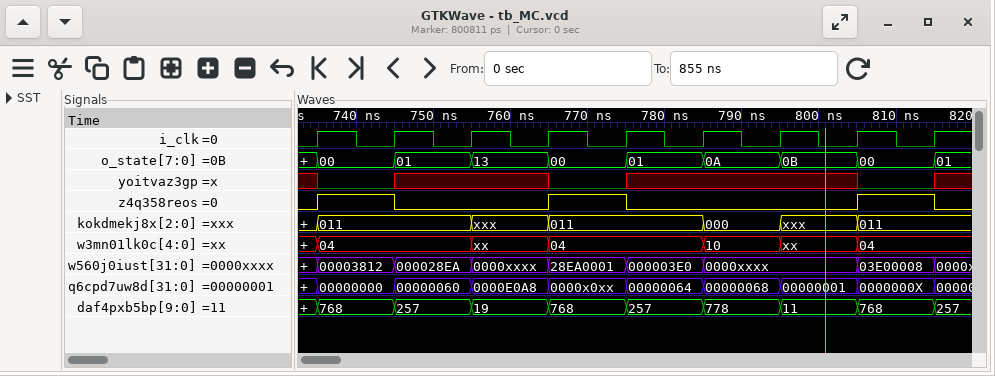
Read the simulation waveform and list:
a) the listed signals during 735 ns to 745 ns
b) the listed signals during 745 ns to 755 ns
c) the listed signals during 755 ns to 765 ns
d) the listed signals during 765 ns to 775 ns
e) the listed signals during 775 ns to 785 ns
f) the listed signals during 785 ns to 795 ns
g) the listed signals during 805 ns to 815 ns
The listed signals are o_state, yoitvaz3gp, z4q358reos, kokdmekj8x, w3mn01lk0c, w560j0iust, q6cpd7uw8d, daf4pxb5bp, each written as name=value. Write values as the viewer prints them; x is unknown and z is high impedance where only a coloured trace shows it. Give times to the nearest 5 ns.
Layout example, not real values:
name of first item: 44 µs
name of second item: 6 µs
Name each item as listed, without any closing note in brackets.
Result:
the listed signals during 735 ns to 745 ns: o_state=00, yoitvaz3gp=0, z4q358reos=1, kokdmekj8x=011, w3mn01lk0c=04, w560j0iust=00003812, q6cpd7uw8d=00000000, daf4pxb5bp=768
the listed signals during 745 ns to 755 ns: o_state=01, yoitvaz3gp=x, z4q358reos=0, kokdmekj8x=011, w3mn01lk0c=04, w560j0iust=000028EA, q6cpd7uw8d=00000060, daf4pxb5bp=257
the listed signals during 755 ns to 765 ns: o_state=13, yoitvaz3gp=x, z4q358reos=0, kokdmekj8x=xxx, w3mn01lk0c=xx, w560j0iust=0000xxxx, q6cpd7uw8d=0000E0A8, daf4pxb5bp=19
the listed signals during 765 ns to 775 ns: o_state=00, yoitvaz3gp=0, z4q358reos=1, kokdmekj8x=011, w3mn01lk0c=04, w560j0iust=28EA0001, q6cpd7uw8d=0000x0xx, daf4pxb5bp=768
the listed signals during 775 ns to 785 ns: o_state=01, yoitvaz3gp=x, z4q358reos=0, kokdmekj8x=011, w3mn01lk0c=04, w560j0iust=000003E0, q6cpd7uw8d=00000064, daf4pxb5bp=257
the listed signals during 785 ns to 795 ns: o_state=0A, yoitvaz3gp=x, z4q358reos=0, kokdmekj8x=000, w3mn01lk0c=10, w560j0iust=0000xxxx, q6cpd7uw8d=00000068, daf4pxb5bp=778
the listed signals during 805 ns to 815 ns: o_state=00, yoitvaz3gp=0, z4q358reos=1, kokdmekj8x=011, w3mn01lk0c=04, w560j0iust=03E00008, q6cpd7uw8d=0000000X, daf4pxb5bp=768
